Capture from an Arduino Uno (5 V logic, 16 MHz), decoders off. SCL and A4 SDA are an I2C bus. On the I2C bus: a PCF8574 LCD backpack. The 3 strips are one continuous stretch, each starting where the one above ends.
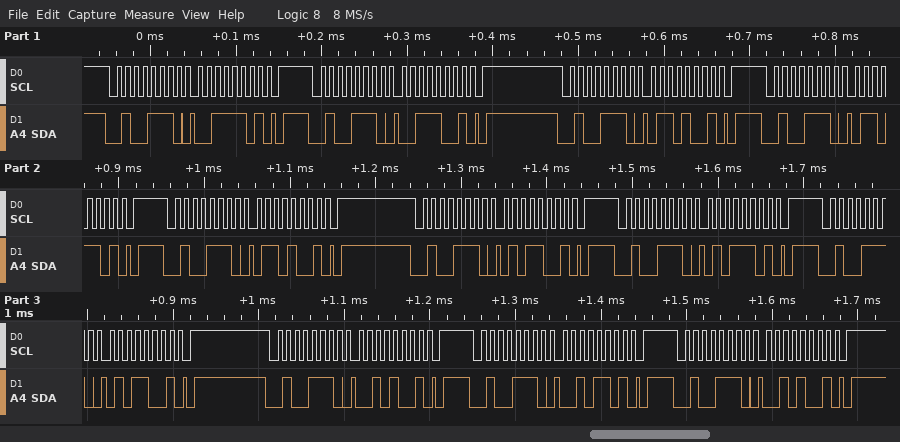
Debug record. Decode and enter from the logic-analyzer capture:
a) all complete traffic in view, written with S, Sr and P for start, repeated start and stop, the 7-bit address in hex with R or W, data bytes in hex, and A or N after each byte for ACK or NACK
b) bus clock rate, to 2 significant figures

S 27W A 3D A P S 27W A 39 A P S 27W A 69 A P S 27W A 6D A P S 27W A 69 A P S 27W A 59 A P S 27W A 5D A P S 27W A 59 A P S 27W A 29 A P S 27W A 2D A P S 27W A 29 A P
100 kHz
